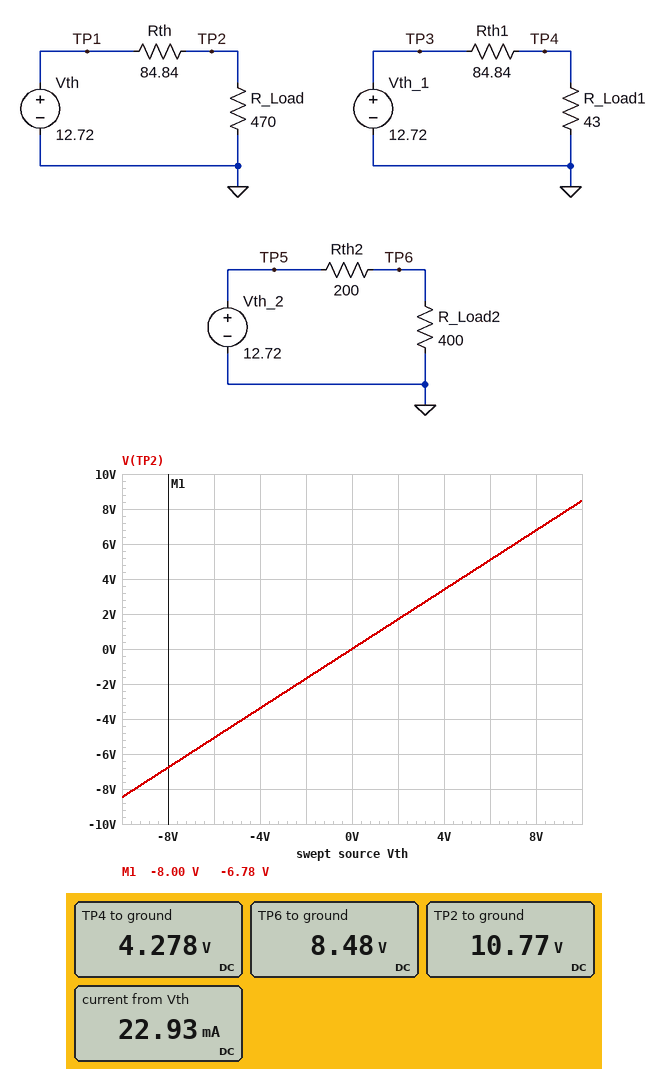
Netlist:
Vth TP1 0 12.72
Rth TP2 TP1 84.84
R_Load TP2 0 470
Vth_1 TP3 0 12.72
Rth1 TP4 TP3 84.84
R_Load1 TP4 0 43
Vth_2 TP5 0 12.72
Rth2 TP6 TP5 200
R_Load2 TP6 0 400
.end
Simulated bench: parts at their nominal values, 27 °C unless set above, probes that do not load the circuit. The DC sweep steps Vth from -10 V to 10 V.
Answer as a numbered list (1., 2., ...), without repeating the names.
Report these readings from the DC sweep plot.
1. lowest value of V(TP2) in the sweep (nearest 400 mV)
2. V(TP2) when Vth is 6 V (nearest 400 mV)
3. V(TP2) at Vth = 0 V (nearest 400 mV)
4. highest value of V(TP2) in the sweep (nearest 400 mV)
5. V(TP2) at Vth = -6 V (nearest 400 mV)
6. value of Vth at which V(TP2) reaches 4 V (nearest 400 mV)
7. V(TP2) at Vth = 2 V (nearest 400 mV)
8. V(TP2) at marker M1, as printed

1. -8.4 V
2. 5.2 V
3. 0 V
4. 8.4 V
5. -5.2 V
6. 4.8 V
7. 1.6 V
8. -6.78 V
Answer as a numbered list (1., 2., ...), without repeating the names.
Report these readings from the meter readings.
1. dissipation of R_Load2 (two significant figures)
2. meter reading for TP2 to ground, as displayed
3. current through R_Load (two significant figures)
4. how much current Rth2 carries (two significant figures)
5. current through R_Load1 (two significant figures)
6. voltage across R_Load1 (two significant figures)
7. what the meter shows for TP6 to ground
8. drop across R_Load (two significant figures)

1. 180 mW
2. 10.77 V
3. 23 mA
4. 21 mA
5. 99 mA
6. 4.3 V
7. 8.48 V
8. 11 V
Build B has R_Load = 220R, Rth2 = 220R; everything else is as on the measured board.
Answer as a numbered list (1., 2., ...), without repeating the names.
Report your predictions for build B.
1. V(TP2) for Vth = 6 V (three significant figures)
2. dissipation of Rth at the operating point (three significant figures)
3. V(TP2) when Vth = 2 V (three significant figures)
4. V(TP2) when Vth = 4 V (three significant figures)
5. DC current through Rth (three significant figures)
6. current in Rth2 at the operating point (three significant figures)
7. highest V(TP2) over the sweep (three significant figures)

1. 4.33 V
2. 148 mW
3. 1.44 V
4. 2.89 V
5. 41.7 mA
6. 20.5 mA
7. 7.22 V
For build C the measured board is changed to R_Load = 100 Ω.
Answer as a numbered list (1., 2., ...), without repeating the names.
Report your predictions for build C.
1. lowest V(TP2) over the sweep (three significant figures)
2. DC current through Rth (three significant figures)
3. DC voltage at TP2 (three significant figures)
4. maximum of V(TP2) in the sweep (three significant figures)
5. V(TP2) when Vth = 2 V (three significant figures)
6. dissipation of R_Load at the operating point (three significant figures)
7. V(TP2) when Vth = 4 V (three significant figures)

1. -5.41 V
2. 68.8 mA
3. 6.88 V
4. 5.41 V
5. 1.08 V
6. 474 mW
7. 2.16 V
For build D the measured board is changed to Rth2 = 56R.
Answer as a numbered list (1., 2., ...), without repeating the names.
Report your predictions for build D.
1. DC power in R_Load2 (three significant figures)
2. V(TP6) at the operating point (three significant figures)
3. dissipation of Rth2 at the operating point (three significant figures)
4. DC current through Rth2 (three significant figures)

1. 311 mW
2. 11.2 V
3. 43.6 mW
4. 27.9 mA
